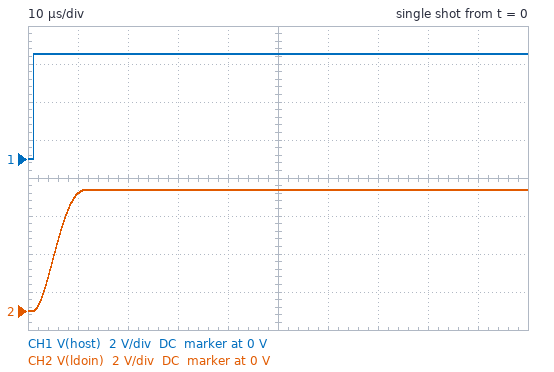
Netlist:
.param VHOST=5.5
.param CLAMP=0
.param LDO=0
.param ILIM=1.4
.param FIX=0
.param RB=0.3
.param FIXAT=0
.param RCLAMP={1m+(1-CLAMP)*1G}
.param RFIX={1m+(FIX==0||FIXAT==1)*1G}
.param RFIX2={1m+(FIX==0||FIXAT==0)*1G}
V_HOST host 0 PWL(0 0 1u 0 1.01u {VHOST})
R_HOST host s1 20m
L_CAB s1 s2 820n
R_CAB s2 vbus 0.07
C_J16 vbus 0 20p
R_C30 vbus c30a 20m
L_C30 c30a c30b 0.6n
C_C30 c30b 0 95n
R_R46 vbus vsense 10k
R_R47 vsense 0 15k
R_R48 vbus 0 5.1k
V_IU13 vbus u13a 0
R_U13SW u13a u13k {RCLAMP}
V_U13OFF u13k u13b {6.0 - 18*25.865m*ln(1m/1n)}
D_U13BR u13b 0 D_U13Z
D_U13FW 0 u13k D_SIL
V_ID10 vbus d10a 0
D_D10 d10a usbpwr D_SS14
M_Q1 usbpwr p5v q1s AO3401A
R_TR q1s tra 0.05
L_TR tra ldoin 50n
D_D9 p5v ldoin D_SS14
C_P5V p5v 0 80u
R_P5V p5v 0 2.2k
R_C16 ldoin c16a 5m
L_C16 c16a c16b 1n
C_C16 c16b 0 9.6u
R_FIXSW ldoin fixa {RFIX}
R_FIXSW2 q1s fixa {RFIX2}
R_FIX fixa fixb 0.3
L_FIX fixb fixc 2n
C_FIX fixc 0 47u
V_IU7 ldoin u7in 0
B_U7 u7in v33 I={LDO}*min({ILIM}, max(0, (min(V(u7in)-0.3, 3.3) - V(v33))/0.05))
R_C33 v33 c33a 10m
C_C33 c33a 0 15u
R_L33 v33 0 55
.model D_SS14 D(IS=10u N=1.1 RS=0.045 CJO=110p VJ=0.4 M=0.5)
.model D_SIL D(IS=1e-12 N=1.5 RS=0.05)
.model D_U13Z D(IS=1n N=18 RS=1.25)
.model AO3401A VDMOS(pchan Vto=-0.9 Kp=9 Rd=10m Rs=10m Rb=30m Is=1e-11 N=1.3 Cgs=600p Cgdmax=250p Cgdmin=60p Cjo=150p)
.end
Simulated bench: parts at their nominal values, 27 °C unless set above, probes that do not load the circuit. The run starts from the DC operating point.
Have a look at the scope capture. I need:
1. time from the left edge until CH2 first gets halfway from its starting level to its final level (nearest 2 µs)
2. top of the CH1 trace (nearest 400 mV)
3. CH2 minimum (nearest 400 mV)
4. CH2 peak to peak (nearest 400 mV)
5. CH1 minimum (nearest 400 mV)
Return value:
6 µs
5.6 V
0 V
6.4 V
0 V
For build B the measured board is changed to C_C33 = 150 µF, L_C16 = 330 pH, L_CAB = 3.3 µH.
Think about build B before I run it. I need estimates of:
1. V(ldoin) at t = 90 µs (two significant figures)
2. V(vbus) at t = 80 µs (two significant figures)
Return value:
7.7 V
6.3 V
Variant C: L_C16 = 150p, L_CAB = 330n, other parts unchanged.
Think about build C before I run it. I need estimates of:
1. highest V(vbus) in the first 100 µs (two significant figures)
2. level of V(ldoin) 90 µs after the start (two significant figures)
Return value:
6.0 V
5.6 V
